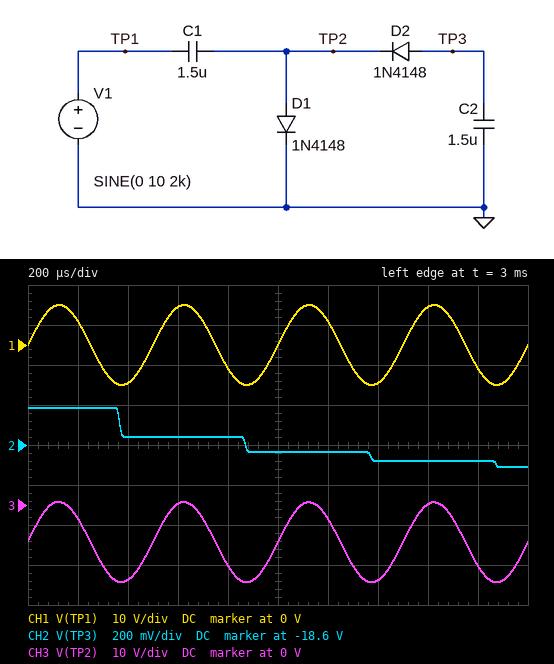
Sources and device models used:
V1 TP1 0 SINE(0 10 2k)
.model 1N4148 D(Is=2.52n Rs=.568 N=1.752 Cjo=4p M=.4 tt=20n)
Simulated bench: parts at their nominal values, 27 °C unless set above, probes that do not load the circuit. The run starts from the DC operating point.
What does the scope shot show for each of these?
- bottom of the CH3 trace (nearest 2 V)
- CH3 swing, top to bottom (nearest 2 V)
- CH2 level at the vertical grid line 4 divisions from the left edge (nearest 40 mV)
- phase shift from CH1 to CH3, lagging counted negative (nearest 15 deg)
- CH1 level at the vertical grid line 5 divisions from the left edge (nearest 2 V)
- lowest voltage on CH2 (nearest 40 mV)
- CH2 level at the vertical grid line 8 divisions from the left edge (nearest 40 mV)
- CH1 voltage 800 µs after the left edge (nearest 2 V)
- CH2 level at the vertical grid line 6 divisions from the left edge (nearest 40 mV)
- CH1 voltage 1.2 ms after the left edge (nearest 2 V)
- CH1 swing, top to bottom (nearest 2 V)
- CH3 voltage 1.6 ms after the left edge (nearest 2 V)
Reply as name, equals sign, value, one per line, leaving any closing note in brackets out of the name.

bottom of the CH3 trace = -20 V
CH3 swing, top to bottom = 20 V
CH2 level at the vertical grid line 4 divisions from the left edge = -18.56 V
phase shift from CH1 to CH3, lagging counted negative = 0 deg
CH1 level at the vertical grid line 5 divisions from the left edge = 0 V
lowest voltage on CH2 = -18.72 V
CH2 level at the vertical grid line 8 divisions from the left edge = -18.68 V
CH1 voltage 800 µs after the left edge = -6 V
CH2 level at the vertical grid line 6 divisions from the left edge = -18.64 V
CH1 voltage 1.2 ms after the left edge = 6 V
CH1 swing, top to bottom = 20 V
CH3 voltage 1.6 ms after the left edge = 0 V
